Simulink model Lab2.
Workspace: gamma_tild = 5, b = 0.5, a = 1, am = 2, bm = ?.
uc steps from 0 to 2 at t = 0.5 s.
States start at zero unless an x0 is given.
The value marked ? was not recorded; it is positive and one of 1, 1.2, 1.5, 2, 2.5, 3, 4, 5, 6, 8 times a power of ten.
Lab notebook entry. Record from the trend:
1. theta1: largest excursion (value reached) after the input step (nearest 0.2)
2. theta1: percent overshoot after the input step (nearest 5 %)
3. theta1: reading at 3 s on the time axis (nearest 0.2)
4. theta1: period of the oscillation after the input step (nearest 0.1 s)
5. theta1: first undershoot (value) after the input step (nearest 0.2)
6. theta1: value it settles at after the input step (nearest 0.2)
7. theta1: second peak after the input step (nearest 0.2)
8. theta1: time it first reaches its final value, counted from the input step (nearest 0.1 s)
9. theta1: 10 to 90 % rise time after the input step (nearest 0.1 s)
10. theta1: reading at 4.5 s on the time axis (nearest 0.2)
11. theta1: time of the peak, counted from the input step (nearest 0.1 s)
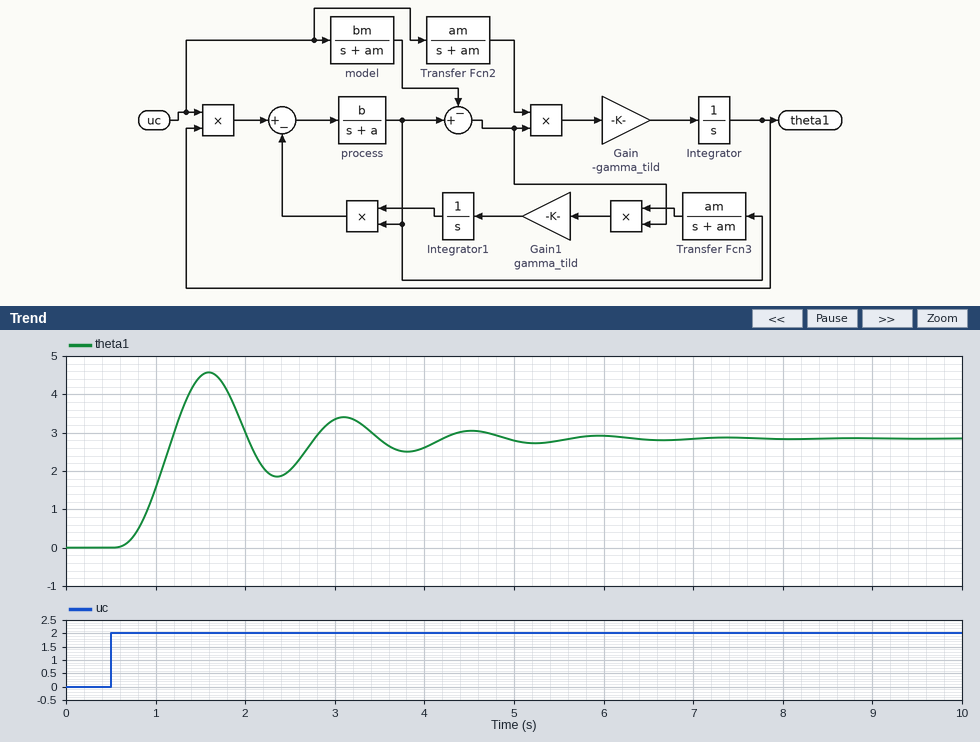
4.6
60 %
3.4
1.5 s
1.8
2.8
3.4
0.7 s
0.4 s
3.0
1.1 s
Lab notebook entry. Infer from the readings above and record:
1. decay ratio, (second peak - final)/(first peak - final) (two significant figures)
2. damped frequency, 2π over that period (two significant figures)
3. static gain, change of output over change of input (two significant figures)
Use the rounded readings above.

0.33
4.2 rad/s
1.4
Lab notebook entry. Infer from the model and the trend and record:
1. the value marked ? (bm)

2
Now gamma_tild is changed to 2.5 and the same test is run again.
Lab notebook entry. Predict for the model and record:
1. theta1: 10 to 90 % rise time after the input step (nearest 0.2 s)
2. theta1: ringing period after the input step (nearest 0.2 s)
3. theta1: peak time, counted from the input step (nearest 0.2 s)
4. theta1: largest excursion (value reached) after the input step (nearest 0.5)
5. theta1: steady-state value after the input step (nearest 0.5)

0.6 s
2.0 s
1.4 s
4.0
2.5
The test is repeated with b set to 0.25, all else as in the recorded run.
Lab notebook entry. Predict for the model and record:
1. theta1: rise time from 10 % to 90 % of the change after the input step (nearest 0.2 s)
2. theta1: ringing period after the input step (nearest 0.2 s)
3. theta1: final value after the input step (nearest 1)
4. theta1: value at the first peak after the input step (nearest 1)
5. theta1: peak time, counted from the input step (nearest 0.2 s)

0.6 s
2.0 s
5
8
1.4 s
